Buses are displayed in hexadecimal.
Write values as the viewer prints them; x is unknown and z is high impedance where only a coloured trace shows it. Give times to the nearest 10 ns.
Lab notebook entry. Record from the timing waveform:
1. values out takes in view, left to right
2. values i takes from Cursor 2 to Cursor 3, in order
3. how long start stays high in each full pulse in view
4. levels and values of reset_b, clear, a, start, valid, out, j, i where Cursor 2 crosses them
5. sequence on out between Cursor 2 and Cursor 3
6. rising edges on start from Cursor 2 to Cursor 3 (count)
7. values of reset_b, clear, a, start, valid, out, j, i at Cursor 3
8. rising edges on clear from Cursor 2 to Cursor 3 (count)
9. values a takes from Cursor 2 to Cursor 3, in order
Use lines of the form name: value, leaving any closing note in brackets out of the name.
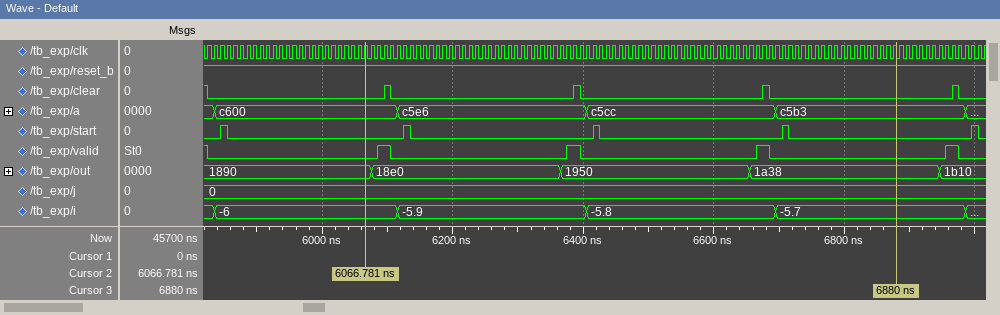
values out takes in view, left to right: 1890, 18e0, 1950, 1a38, 1b10
values i takes from Cursor 2 to Cursor 3, in order: -6, -5.9, -5.8, -5.7
how long start stays high in each full pulse in view: 10 ns, 10 ns, 10 ns, 10 ns, 10 ns
levels and values of reset_b, clear, a, start, valid, out, j, i where Cursor 2 crosses them: reset_b=1, clear=0, a=c600, start=0, valid=0, out=1890, j=0, i=-6
sequence on out between Cursor 2 and Cursor 3: 1890, 18e0, 1950, 1a38
rising edges on start from Cursor 2 to Cursor 3: 3
values of reset_b, clear, a, start, valid, out, j, i at Cursor 3: reset_b=1, clear=0, a=c5b3, start=0, valid=0, out=1a38, j=0, i=-5.7
rising edges on clear from Cursor 2 to Cursor 3: 3
values a takes from Cursor 2 to Cursor 3, in order: c600, c5e6, c5cc, c5b3
